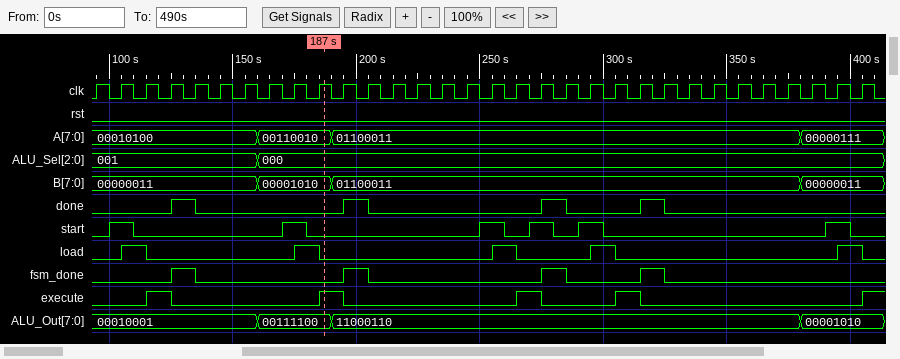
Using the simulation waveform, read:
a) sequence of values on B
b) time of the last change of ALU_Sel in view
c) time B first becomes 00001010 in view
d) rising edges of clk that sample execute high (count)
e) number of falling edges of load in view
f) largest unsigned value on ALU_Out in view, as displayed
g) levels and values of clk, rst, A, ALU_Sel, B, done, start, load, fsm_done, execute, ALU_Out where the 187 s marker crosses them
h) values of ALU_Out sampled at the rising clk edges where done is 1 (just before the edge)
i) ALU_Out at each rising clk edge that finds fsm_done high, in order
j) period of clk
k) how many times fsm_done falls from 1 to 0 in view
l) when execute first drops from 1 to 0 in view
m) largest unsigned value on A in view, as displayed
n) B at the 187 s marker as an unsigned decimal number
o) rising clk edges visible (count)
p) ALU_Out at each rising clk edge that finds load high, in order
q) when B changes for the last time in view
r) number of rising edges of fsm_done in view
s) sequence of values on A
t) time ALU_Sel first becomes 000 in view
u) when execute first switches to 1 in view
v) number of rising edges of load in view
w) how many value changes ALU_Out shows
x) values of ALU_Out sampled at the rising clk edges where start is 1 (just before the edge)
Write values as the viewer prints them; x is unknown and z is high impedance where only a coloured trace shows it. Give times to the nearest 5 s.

00000011, 00001010, 01100011, 00000011
160 s
160 s
4
5
11000110
clk=1, rst=0, A=00110010, ALU_Sel=000, B=00001010, done=0, start=0, load=0, fsm_done=0, execute=1, ALU_Out=00111100
00010001, 11000110, 11000110, 11000110
00010001, 11000110, 11000110, 11000110
10 s
4
125 s
01100011
10
32
00010001, 00111100, 11000110, 11000110, 00001010
380 s
4
00010100, 00110010, 01100011, 00000111
160 s
115 s
5
3
00010001, 00111100, 11000110, 11000110, 11000110, 00001010
